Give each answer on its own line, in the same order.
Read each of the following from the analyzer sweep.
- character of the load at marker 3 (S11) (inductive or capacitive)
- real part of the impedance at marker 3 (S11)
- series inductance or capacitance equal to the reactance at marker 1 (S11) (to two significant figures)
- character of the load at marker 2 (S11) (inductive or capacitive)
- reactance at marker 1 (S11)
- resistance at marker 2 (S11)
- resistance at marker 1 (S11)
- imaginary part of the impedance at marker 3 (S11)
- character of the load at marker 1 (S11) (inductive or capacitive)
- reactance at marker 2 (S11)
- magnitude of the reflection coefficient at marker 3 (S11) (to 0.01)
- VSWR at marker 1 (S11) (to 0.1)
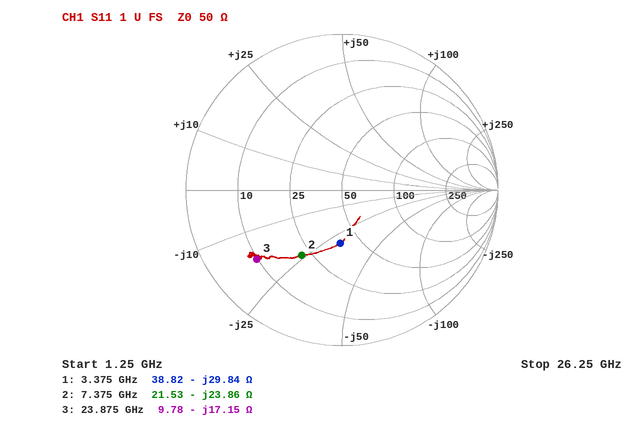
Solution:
capacitive
9.78 Ω
1.6 pF
capacitive
-29.84 Ω
21.53 Ω
38.82 Ω
-17.15 Ω
capacitive
-23.86 Ω
0.70
2.0
